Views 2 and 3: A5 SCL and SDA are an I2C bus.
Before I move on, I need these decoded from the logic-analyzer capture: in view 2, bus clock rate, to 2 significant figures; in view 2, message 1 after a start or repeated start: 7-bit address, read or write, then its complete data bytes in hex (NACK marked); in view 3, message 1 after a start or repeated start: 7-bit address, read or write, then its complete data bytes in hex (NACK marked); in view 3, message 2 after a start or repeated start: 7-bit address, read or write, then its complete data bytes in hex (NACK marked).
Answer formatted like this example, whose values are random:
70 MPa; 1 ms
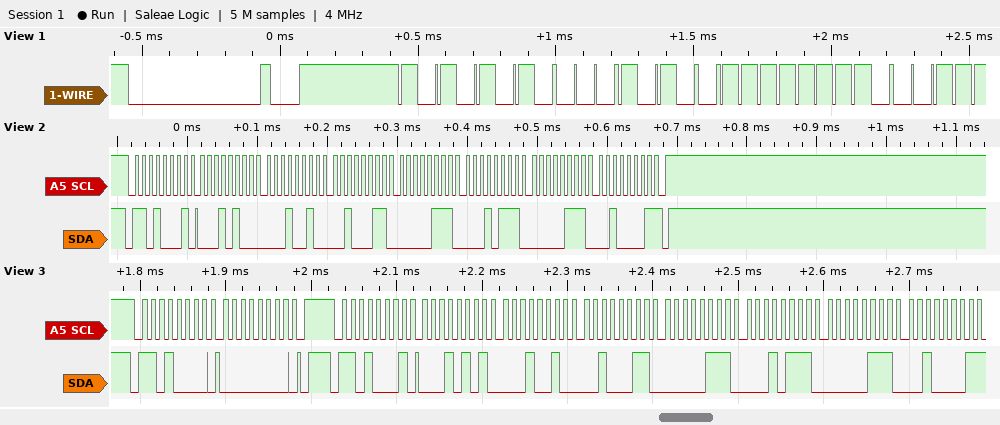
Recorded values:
100 kHz; 0x68 read: 14 12 23 07 17 07 21 NACK; 0x68 write: 00; 0x68 read: 15 12 23 07 17 07 21 NACK
